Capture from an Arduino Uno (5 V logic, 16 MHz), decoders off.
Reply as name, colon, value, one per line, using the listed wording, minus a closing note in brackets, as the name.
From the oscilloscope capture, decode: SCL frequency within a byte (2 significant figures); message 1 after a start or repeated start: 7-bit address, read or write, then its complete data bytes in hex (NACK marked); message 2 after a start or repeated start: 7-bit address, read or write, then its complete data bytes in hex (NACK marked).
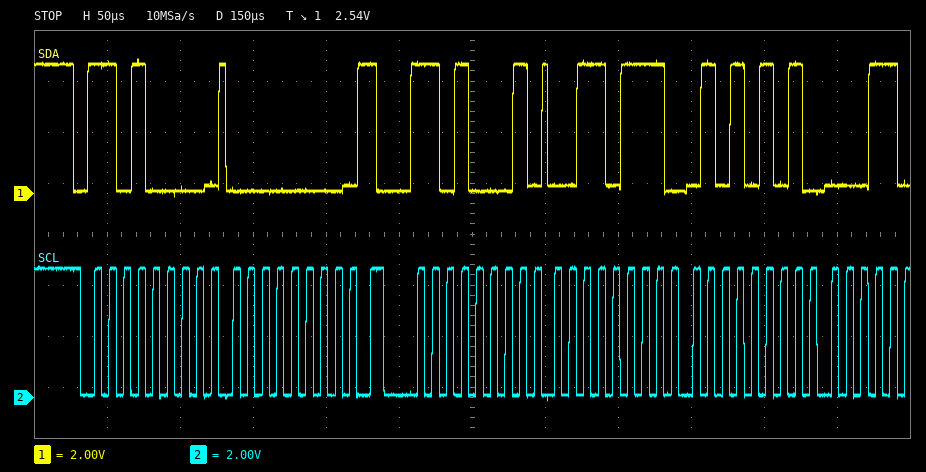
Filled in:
SCL frequency within a byte: 100 kHz
message 1 after a start or repeated start: 7-bit address, read or write, then its complete data bytes in hex: 0x68 write: 00
message 2 after a start or repeated start: 7-bit address, read or write, then its complete data bytes in hex: 0x68 read: 37 55
